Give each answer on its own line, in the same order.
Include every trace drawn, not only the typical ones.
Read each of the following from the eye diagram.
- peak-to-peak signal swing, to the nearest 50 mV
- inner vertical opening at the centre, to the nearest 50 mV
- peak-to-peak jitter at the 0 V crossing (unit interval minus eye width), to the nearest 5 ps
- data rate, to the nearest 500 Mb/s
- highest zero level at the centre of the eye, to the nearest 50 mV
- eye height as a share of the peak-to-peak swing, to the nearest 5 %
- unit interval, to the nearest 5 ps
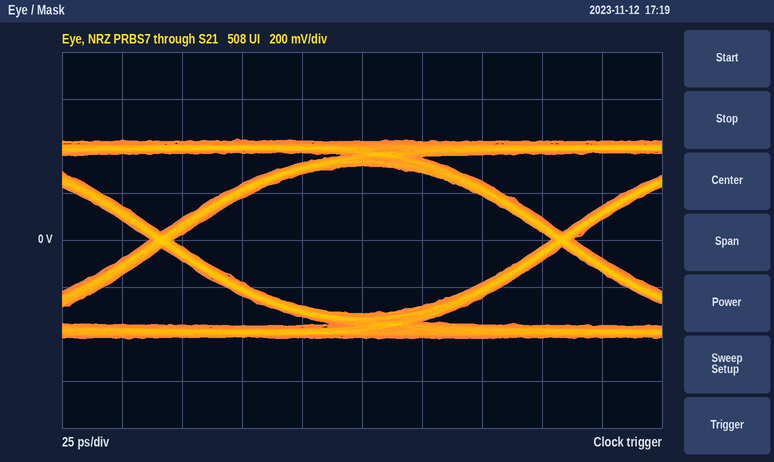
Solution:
850 mV
650 mV
10 ps
6.0 Gb/s
-300 mV
75 %
165 ps
